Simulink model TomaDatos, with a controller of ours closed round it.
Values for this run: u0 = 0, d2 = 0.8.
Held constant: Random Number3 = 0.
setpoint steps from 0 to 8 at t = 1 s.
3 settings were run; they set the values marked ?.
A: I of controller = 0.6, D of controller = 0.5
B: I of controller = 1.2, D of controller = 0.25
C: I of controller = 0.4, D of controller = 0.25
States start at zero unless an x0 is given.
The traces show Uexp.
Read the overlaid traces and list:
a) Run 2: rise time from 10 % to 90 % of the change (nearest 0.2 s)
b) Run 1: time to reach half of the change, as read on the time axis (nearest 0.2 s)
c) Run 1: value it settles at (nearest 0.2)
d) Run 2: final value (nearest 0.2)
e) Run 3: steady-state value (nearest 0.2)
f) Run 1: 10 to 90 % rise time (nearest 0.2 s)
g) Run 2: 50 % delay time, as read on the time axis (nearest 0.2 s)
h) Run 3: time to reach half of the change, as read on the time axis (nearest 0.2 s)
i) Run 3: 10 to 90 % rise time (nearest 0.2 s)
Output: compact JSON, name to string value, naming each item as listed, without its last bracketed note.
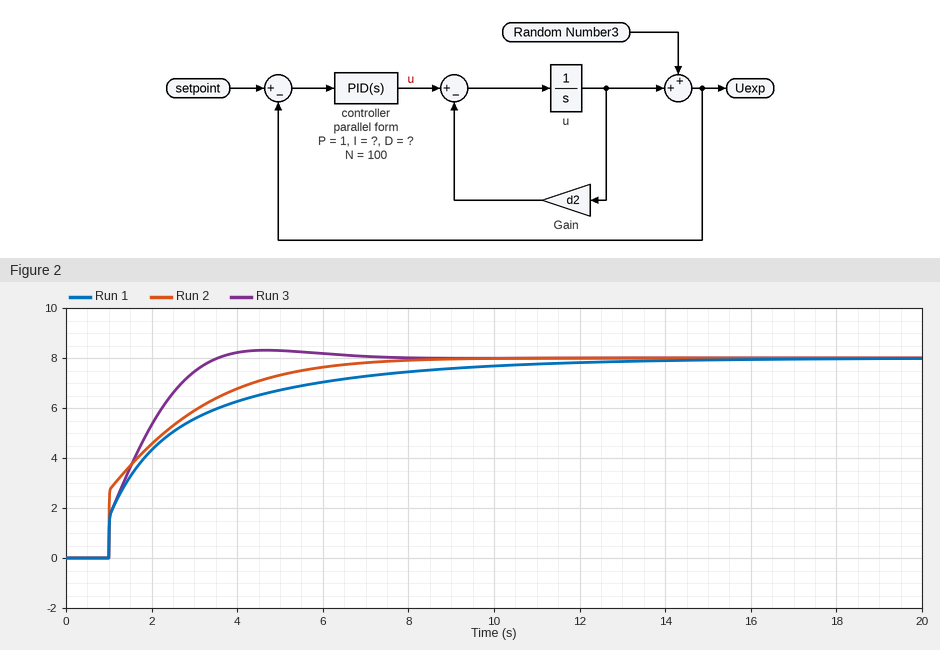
{"Run 2: rise time from 10 % to 90 % of the change": "3.8 s", "Run 1: time to reach half of the change, as read on the time axis": "1.8 s", "Run 1: value it settles at": "8.0", "Run 2: final value": "8.0", "Run 3: steady-state value": "8.0", "Run 1: 10 to 90 % rise time": "5.6 s", "Run 2: 50 % delay time, as read on the time axis": "1.6 s", "Run 3: time to reach half of the change, as read on the time axis": "1.6 s", "Run 3: 10 to 90 % rise time": "1.8 s"}
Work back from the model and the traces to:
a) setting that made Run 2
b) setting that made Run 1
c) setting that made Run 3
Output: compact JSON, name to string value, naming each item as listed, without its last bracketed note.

{"setting that made Run 2": "A", "setting that made Run 1": "C", "setting that made Run 3": "B"}
